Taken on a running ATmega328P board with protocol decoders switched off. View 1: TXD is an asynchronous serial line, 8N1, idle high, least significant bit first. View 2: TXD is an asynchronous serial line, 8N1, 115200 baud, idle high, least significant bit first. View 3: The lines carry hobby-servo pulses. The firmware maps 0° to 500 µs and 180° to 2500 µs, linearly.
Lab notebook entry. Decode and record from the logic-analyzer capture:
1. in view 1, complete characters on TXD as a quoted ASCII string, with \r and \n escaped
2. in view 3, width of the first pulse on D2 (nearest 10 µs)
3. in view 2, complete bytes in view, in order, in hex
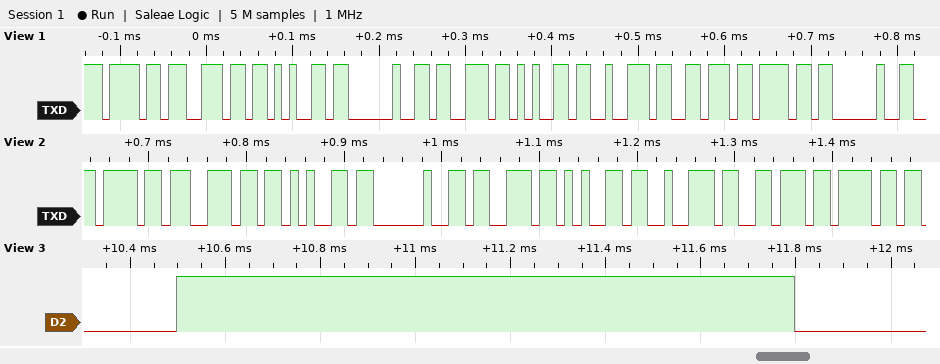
"one servo "
1300 µs
6F 6E 65 20 73 65 72 76 6F
